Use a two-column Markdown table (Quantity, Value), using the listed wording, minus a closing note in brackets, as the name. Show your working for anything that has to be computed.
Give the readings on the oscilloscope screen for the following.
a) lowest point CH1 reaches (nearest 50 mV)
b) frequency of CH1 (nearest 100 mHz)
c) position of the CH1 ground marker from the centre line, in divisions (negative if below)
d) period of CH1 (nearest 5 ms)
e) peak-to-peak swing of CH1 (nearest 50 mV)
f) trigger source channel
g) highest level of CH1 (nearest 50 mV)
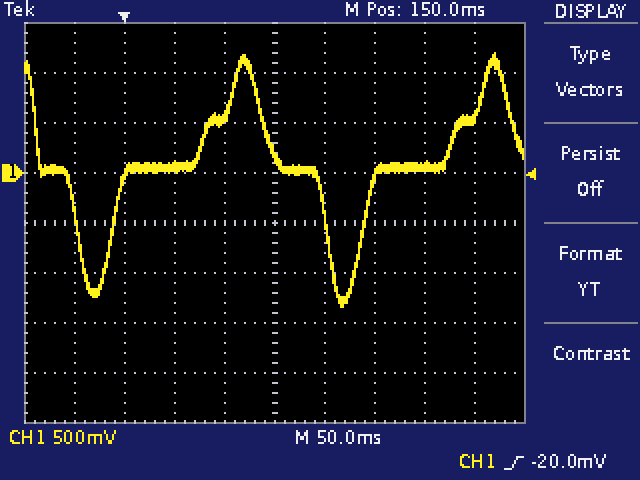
| Quantity | Value |
|---|---|
| lowest point CH1 reaches | -1.35 V |
| frequency of CH1 | 1 / 250 ms ≈ 4.0 Hz |
| position of the CH1 ground marker from the centre line, in divisions | +1.0 div |
| period of CH1 | 250 ms |
| peak-to-peak swing of CH1 | 1.20 V − (-1.35 V) = 2.55 V |
| trigger source channel | CH1 |
| highest level of CH1 | 1.20 V |
